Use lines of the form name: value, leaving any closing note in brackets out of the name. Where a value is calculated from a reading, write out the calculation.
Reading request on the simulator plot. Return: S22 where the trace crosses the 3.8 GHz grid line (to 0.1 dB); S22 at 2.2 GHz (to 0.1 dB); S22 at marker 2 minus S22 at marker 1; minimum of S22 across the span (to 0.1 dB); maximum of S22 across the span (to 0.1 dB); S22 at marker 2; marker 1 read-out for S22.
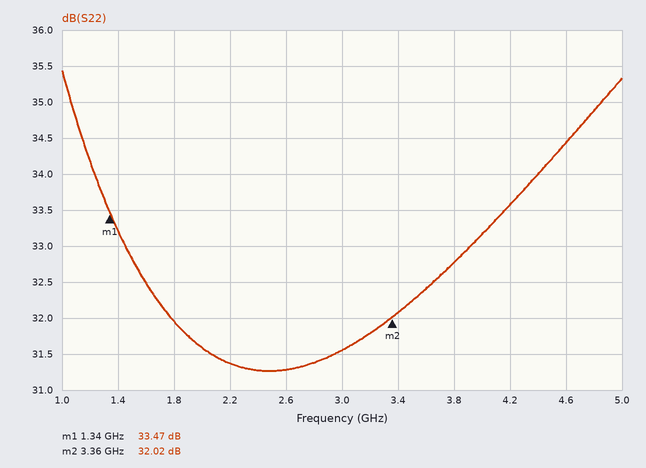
S22 where the trace crosses the 3.8 GHz grid line: 32.8 dB
S22 at 2.2 GHz: 31.4 dB
S22 at marker 2 minus S22 at marker 1: 32.02 − (33.47) = -1.45 dB
minimum of S22 across the span: 31.3 dB
maximum of S22 across the span: 35.4 dB
S22 at marker 2: 32.02 dB
marker 1 read-out for S22: 33.47 dB
